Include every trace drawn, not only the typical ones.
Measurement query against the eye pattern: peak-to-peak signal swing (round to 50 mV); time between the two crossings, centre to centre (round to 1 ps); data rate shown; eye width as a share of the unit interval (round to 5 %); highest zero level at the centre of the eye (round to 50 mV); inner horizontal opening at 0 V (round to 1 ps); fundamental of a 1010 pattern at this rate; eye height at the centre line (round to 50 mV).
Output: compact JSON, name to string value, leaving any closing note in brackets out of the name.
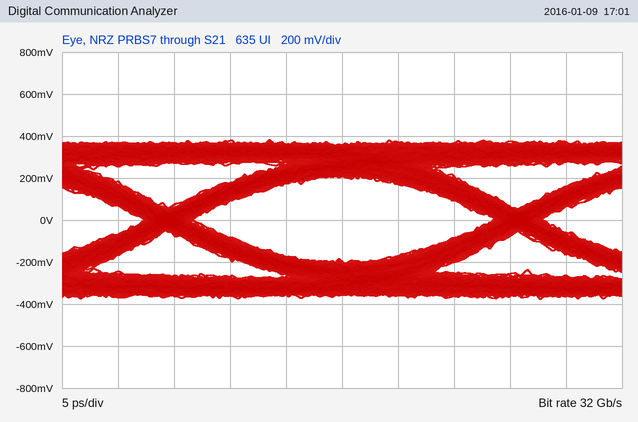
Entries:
{"peak-to-peak signal swing": "750 mV", "time between the two crossings, centre to centre": "31 ps", "data rate shown": "32 Gb/s", "eye width as a share of the unit interval": "85 %", "highest zero level at the centre of the eye": "-200 mV", "inner horizontal opening at 0 V": "27 ps", "fundamental of a 1010 pattern at this rate": "16 GHz", "eye height at the centre line": "400 mV"}
